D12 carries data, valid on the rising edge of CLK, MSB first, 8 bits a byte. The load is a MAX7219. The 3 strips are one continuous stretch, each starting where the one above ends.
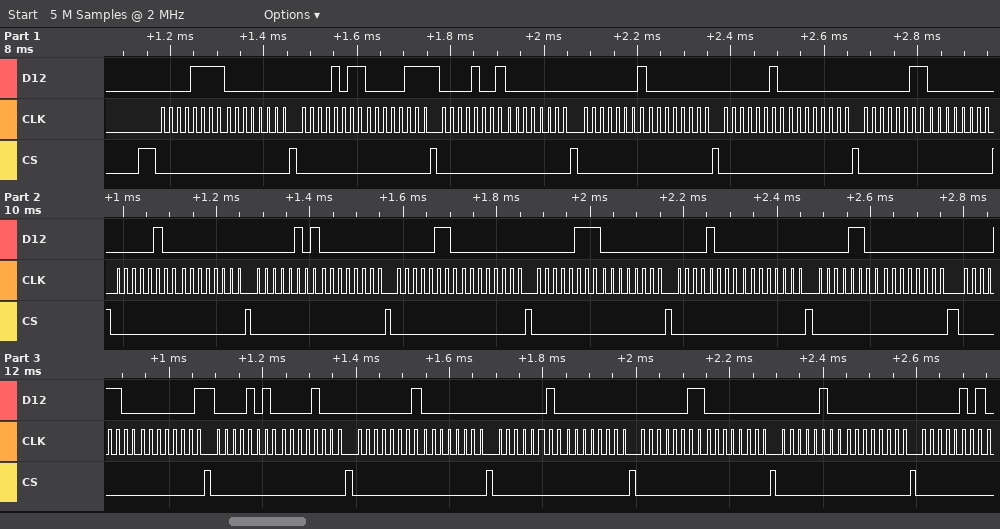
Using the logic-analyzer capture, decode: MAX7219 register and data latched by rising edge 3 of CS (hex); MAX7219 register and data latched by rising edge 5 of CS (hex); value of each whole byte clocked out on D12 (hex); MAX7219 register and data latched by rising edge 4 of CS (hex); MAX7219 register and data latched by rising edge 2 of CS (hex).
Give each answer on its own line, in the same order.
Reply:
register 0xB, data 0x07
register 0x1, data 0x00
0F 00 0B 07 09 00 01 00 02 00 03 00 04 00 05 00 06 00 07 00 08 00 0C 00 0C 01 0A 08 01 00 02 00 03 00 04 00 05
register 0x9, data 0x00
register 0xF, data 0x00
